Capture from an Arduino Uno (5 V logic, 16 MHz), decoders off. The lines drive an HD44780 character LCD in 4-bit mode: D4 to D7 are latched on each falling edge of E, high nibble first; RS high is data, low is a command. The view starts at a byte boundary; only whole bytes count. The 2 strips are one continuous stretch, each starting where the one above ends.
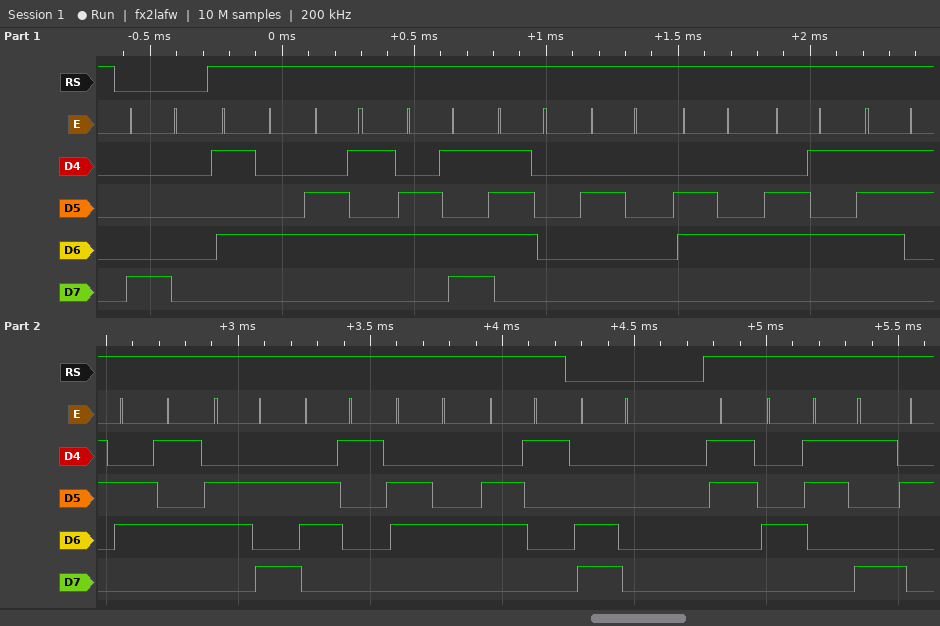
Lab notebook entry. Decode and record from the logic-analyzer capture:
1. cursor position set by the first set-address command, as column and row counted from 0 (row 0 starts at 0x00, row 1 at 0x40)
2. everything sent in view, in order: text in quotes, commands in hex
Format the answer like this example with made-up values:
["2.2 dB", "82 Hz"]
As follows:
["column 0, row 0", "0x80 \"Temp desejada\" 0xC0 \"49\""]
